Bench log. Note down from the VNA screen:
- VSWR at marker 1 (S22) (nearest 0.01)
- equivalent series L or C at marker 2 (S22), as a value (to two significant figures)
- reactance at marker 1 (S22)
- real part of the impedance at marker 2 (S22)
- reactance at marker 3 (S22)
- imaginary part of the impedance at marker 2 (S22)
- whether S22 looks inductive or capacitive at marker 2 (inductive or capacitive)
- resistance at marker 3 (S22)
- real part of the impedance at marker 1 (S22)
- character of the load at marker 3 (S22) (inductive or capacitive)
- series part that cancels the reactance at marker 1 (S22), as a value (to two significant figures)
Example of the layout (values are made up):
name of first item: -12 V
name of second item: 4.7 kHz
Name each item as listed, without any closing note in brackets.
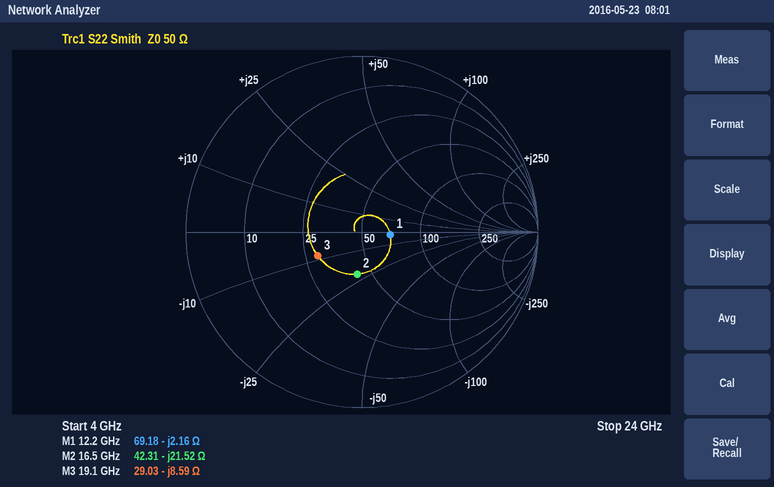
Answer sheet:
VSWR at marker 1 (S22): 1.39
equivalent series L or C at marker 2 (S22), as a value: 450 fF
reactance at marker 1: -2.16 Ω
real part of the impedance at marker 2: 42.31 Ω
reactance at marker 3: -8.59 Ω
imaginary part of the impedance at marker 2: -21.52 Ω
whether S22 looks inductive or capacitive at marker 2: capacitive
resistance at marker 3: 29.03 Ω
real part of the impedance at marker 1: 69.18 Ω
character of the load at marker 3 (S22): capacitive
series part that cancels the reactance at marker 1 (S22), as a value: 28 pH
